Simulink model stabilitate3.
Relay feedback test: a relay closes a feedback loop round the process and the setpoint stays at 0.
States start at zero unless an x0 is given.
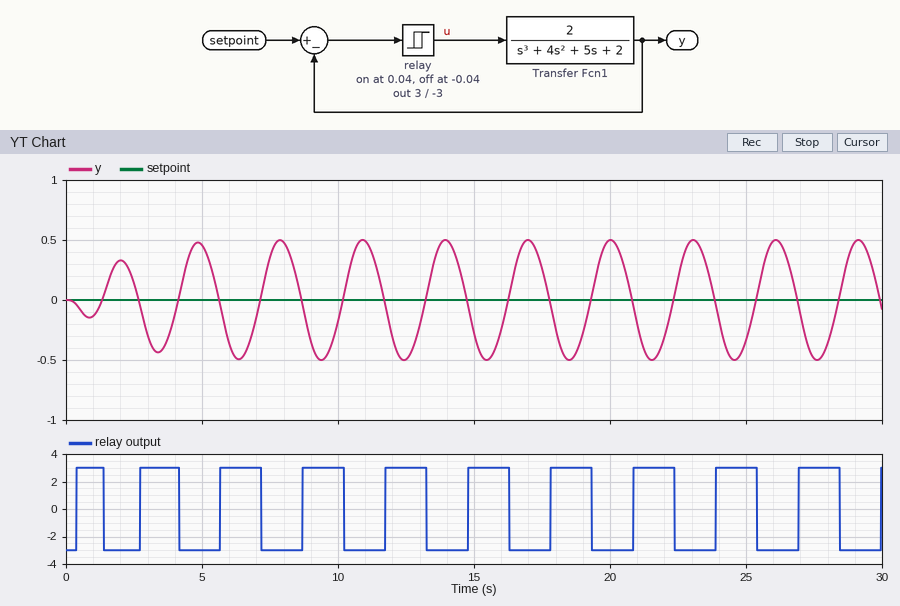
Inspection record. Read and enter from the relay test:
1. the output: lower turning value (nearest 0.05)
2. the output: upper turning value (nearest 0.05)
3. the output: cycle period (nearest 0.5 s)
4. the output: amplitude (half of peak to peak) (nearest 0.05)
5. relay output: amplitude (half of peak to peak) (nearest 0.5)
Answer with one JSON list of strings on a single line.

["-0.50", "0.50", "3.0 s", "0.50", "3.0"]
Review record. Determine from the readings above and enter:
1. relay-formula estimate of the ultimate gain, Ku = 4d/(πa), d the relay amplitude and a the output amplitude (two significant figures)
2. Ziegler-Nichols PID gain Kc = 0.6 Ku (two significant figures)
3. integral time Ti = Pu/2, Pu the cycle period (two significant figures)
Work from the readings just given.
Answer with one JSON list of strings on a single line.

["7.6", "4.6", "1.5 s"]
